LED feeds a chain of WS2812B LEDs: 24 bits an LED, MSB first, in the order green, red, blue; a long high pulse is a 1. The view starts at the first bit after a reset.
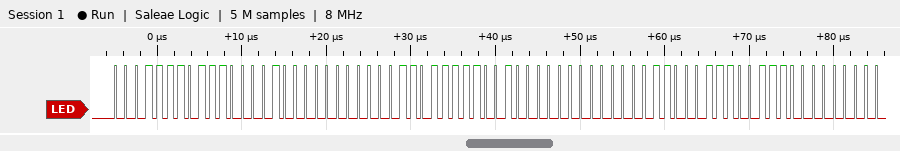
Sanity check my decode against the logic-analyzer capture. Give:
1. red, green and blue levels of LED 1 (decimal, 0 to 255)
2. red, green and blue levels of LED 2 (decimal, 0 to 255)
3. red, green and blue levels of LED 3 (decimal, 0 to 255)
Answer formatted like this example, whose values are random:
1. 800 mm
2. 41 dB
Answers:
1. 225, 30, 0
2. 228, 27, 0
3. 231, 24, 0
